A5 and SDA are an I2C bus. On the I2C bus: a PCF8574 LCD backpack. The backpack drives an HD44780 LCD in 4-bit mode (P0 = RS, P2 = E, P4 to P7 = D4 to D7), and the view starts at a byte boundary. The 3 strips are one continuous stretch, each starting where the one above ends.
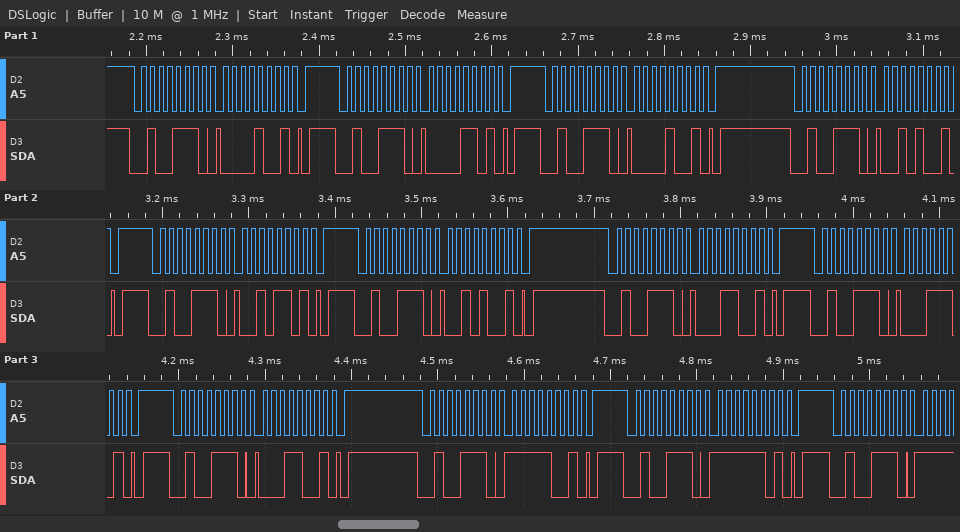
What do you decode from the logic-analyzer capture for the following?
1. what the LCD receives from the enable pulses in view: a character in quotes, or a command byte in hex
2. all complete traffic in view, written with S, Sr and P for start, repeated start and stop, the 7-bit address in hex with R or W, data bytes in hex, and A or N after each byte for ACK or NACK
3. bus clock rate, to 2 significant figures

data 0x02
S 27W A 09 A P S 27W A 0D A P S 27W A 09 A P S 27W A 29 A P S 27W A 2D A P S 27W A 29 A P S 27W A 19 A P S 27W A 1D A P S 27W A 19 A P S 27W A F9 A P S 27W A FD A P S 27W A
100 kHz
